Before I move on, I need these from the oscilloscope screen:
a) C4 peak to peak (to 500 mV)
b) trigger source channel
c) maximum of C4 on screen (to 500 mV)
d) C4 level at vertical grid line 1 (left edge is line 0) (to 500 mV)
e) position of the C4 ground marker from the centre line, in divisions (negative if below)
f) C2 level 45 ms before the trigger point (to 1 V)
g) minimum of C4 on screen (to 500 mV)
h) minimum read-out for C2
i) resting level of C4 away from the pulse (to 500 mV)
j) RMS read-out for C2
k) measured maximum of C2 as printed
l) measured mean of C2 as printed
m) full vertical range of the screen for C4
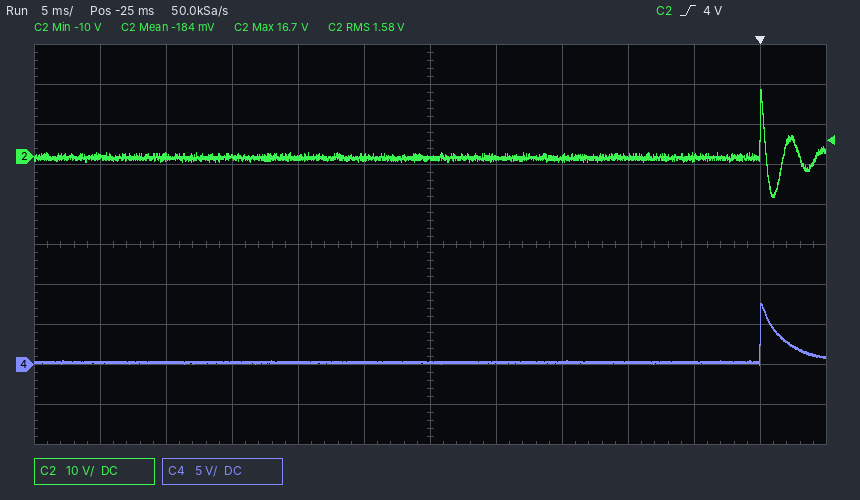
7.5 V
C2
7.5 V
500 mV
-3.0 div
0 V
0.0 V
-10 V
500 mV
1.58 V
16.7 V
-184 mV
50 V
